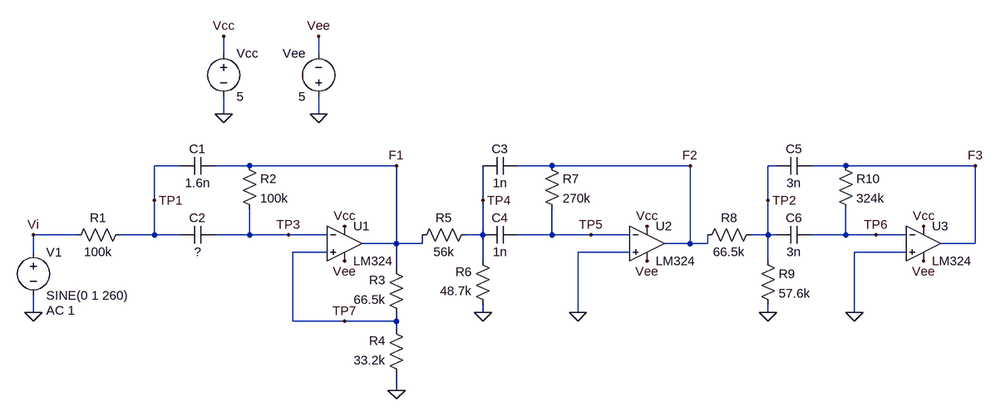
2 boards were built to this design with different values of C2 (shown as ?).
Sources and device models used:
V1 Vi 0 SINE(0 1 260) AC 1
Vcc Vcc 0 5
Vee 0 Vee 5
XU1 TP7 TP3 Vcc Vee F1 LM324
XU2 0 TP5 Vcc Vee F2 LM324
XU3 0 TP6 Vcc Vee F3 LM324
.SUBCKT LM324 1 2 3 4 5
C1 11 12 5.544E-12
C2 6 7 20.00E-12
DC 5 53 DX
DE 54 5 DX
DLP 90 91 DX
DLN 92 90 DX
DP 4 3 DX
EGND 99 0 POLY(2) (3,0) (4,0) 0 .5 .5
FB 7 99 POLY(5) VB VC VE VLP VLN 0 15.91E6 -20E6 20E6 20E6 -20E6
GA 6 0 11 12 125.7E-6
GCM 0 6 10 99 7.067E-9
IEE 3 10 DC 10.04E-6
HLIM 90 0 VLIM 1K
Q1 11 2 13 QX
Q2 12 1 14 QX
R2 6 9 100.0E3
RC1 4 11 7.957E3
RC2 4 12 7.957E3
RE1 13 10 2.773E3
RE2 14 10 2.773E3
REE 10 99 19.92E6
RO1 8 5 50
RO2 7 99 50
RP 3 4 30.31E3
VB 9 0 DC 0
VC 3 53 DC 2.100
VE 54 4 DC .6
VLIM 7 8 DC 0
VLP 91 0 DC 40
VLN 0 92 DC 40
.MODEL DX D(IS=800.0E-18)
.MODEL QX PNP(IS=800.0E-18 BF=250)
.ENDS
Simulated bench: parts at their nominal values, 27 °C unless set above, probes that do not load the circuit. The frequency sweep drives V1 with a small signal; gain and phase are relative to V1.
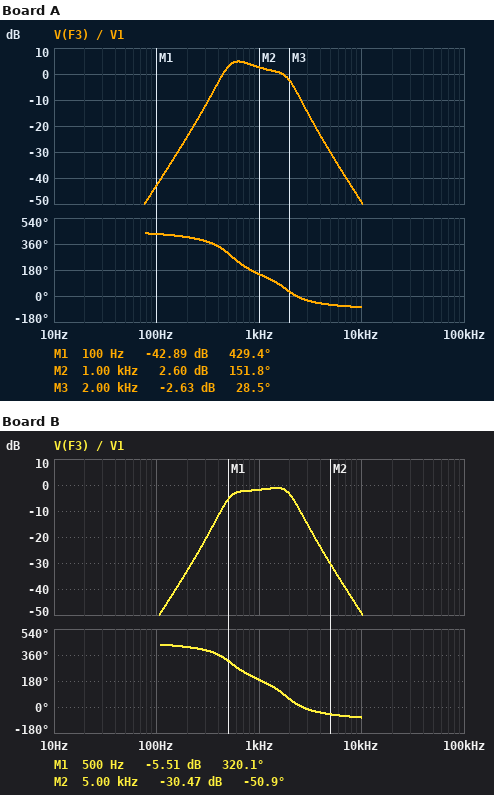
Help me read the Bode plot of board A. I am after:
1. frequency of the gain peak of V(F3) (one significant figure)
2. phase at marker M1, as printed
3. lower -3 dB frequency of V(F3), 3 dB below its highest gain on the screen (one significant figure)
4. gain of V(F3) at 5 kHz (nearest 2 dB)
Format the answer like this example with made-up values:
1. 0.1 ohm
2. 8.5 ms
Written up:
1. 600 Hz
2. 429.4 deg
3. 500 Hz
4. -30 dB
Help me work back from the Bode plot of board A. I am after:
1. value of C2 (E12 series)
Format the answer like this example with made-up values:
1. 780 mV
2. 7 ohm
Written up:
1. 3.3 nF
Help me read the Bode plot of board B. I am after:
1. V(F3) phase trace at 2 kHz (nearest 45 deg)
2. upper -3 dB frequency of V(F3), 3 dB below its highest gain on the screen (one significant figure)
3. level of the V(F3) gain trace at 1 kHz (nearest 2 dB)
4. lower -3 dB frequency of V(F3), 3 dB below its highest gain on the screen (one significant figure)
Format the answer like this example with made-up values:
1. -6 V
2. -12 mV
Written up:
1. 45 deg
2. 2 kHz
3. -2 dB
4. 500 Hz
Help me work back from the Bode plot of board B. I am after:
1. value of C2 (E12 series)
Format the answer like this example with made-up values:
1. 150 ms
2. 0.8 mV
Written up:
1. 1.2 nF
